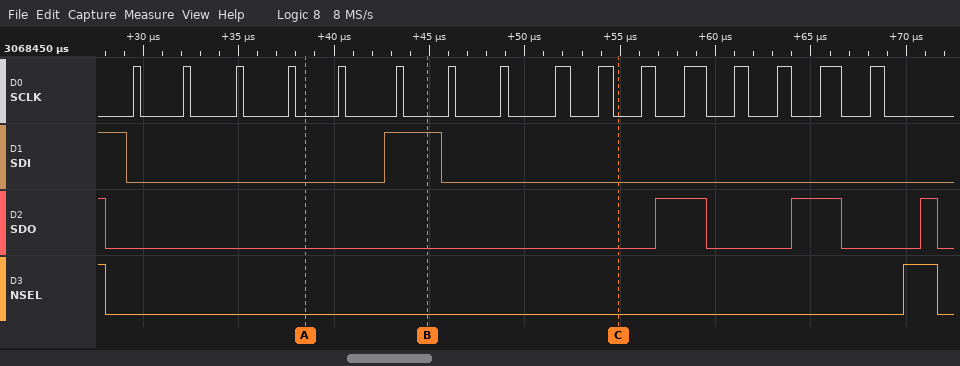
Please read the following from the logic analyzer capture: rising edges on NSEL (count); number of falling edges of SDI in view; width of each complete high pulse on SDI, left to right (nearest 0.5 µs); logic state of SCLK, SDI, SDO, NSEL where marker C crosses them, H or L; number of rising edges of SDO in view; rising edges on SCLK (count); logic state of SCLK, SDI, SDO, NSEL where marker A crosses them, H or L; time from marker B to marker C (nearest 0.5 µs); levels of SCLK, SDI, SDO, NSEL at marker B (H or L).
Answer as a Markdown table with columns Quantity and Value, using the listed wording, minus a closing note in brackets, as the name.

| Quantity | Value |
|---|---|
| rising edges on NSEL | 1 |
| number of falling edges of SDI in view | 2 |
| width of each complete high pulse on SDI, left to right | 3 µs |
| logic state of SCLK, SDI, SDO, NSEL where marker C crosses them, H or L | SCLK=L, SDI=L, SDO=L, NSEL=L |
| number of rising edges of SDO in view | 3 |
| rising edges on SCLK | 16 |
| logic state of SCLK, SDI, SDO, NSEL where marker A crosses them, H or L | SCLK=L, SDI=L, SDO=L, NSEL=L |
| time from marker B to marker C | 10 µs |
| levels of SCLK, SDI, SDO, NSEL at marker B | SCLK=L, SDI=H, SDO=L, NSEL=L |
